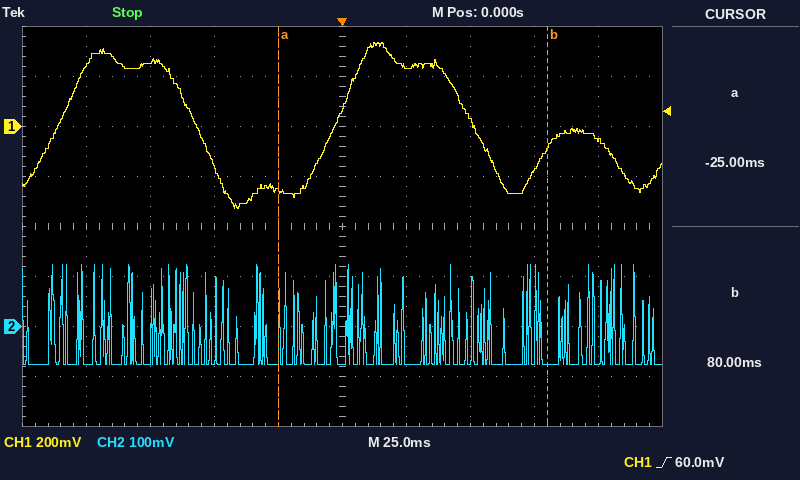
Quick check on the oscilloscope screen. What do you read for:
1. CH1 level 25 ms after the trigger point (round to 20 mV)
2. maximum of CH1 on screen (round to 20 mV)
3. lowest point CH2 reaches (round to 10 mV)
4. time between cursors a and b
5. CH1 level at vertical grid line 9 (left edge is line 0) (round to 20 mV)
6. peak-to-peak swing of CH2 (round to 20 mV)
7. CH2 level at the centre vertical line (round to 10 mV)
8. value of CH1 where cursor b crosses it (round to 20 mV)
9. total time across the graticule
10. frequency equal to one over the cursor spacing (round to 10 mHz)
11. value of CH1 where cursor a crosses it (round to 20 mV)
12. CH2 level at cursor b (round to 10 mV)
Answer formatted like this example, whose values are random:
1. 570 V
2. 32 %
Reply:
1. 240 mV
2. 340 mV
3. -80 mV
4. 105.0 ms
5. -60 mV
6. 200 mV
7. -80 mV
8. -80 mV
9. 250 ms
10. 9.52 Hz
11. -260 mV
12. -80 mV
